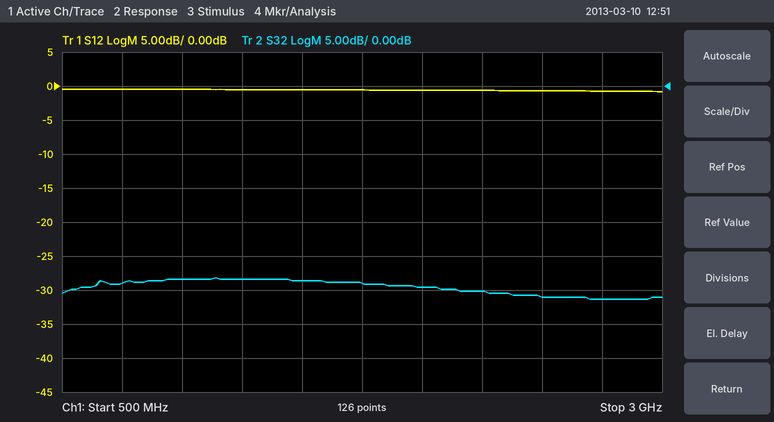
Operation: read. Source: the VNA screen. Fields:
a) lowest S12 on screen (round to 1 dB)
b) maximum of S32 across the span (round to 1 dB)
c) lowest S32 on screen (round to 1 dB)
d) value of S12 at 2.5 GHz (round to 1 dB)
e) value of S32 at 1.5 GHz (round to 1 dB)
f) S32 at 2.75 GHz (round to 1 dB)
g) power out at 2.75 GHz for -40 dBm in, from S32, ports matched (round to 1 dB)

-1 dB
-28 dB
-31 dB
-1 dB
-29 dB
-31 dB
-71 dBm
